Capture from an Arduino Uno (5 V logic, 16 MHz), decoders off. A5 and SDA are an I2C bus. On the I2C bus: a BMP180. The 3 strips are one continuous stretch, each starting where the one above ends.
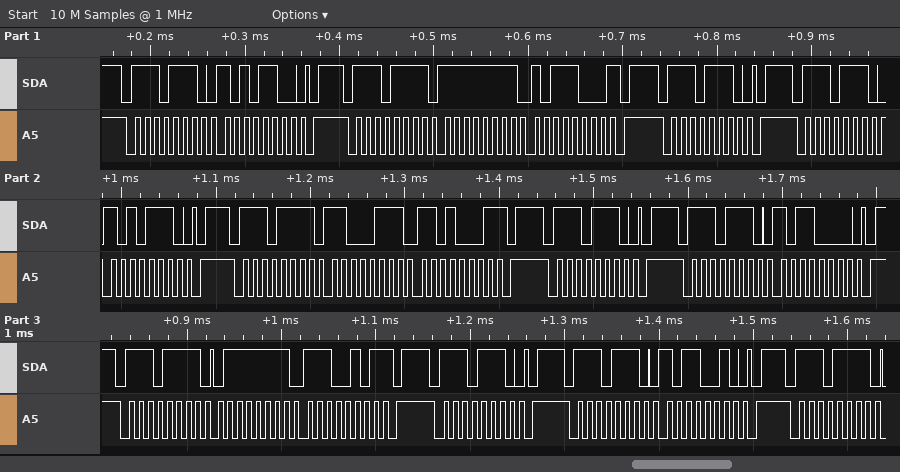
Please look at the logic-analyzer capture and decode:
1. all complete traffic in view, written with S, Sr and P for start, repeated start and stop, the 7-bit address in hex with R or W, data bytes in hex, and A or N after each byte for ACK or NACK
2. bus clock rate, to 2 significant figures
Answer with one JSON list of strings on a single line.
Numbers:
["S 77W A AC A P S 77R A FF A B8 N P S 77W A P S 77W A AE A P S 77R A C7 A D1 N P S 77W A P S 77W A B0 A P S 77R A 7F A E5 N P S 77W A P S 77W A B2 A P S 77R A", "100 kHz"]
